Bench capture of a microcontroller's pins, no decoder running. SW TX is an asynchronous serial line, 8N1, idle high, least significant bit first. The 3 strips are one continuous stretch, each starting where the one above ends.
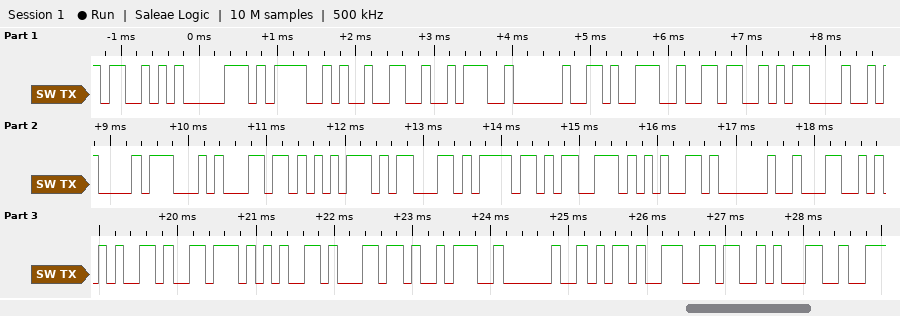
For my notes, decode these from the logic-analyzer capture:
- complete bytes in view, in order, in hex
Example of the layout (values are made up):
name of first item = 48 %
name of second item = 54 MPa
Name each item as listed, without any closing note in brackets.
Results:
complete bytes in view, in order, in hex = 53 70 4F 32 3A 20 39 36 0D 0A 47 6C 75 63 6F 73 65 20 4C 65 76 65 6C 3A 20 2D 36 31
